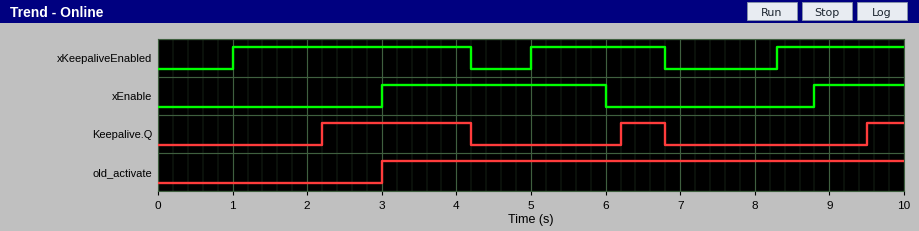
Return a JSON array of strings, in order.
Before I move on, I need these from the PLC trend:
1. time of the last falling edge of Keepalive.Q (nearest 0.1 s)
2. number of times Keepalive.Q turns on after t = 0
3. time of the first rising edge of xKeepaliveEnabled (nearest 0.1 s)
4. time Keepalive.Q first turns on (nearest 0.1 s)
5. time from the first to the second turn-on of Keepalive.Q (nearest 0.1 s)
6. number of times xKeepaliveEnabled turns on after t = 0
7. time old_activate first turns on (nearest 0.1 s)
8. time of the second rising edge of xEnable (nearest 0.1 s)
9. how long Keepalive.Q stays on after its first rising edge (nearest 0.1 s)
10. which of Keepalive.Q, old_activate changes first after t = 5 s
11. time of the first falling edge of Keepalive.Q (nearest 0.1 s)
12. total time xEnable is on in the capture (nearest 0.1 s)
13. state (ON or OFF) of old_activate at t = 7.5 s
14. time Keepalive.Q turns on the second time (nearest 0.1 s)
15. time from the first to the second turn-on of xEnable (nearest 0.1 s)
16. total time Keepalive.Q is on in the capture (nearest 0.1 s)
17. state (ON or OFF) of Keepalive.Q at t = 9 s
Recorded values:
["6.8 s", "3", "1.0 s", "2.2 s", "4.0 s", "3", "3.0 s", "8.8 s", "2.0 s", "Keepalive.Q", "4.2 s", "4.2 s", "ON", "6.2 s", "5.8 s", "3.1 s", "OFF"]
